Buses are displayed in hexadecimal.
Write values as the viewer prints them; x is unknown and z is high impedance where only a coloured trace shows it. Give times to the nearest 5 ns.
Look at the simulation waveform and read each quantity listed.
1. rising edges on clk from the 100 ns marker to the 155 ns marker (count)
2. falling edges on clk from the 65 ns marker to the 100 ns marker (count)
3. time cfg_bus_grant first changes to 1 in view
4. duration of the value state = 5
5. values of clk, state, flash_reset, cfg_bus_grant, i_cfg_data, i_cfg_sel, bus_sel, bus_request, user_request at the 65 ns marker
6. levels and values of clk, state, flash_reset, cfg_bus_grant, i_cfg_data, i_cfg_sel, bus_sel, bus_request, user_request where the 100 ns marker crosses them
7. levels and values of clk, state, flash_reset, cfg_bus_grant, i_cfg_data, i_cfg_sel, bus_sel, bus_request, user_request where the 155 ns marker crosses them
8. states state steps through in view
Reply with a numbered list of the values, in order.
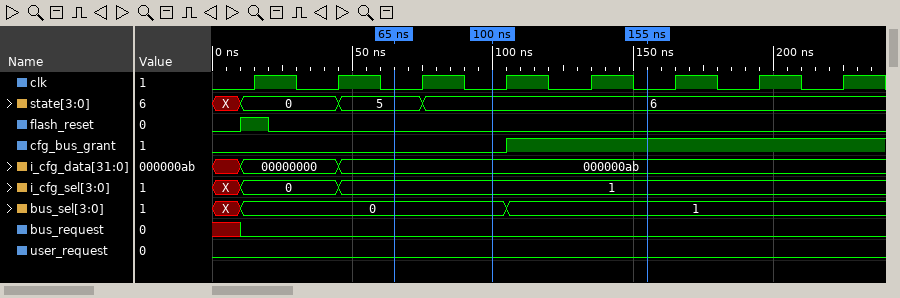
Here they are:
1. 2
2. 1
3. 105 ns
4. 30 ns
5. clk=0, state=5, flash_reset=0, cfg_bus_grant=0, i_cfg_data=000000ab, i_cfg_sel=1, bus_sel=0, bus_request=0, user_request=0
6. clk=0, state=6, flash_reset=0, cfg_bus_grant=0, i_cfg_data=000000ab, i_cfg_sel=1, bus_sel=0, bus_request=0, user_request=0
7. clk=0, state=6, flash_reset=0, cfg_bus_grant=1, i_cfg_data=000000ab, i_cfg_sel=1, bus_sel=1, bus_request=0, user_request=0
8. X, 0, 5, 6
